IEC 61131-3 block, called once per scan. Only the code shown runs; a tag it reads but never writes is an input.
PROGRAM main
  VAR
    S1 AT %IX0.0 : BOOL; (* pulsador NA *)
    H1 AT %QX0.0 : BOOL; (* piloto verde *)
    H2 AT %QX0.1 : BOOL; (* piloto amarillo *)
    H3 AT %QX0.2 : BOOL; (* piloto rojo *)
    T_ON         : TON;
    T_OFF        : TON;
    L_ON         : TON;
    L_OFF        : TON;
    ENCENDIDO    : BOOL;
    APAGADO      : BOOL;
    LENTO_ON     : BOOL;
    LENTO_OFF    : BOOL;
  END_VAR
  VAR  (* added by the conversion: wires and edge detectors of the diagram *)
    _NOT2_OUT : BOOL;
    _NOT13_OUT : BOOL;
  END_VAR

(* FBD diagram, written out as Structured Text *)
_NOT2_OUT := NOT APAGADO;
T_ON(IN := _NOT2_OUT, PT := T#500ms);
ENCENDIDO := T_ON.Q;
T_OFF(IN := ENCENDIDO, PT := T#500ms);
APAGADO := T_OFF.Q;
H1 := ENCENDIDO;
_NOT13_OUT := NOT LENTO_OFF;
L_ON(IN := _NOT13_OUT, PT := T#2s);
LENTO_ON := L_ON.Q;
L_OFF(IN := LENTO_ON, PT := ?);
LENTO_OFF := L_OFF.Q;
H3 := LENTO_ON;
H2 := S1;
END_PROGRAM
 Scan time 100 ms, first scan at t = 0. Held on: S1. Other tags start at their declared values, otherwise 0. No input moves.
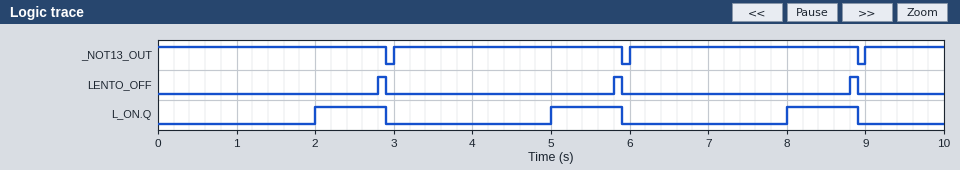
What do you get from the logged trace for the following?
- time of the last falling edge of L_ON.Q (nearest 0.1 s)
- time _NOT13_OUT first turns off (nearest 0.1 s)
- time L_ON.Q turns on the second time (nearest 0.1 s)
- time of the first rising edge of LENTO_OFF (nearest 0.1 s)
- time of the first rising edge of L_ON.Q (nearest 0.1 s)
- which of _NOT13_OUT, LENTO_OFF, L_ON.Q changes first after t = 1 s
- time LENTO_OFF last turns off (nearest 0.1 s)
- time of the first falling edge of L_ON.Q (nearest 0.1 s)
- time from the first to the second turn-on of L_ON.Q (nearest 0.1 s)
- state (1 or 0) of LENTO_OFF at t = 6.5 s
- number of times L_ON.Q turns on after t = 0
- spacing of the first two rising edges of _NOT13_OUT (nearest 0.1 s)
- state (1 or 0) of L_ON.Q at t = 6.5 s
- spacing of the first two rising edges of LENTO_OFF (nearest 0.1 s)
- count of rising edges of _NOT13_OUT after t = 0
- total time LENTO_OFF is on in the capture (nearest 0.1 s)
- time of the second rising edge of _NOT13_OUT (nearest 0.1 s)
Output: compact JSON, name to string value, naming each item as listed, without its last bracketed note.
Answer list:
{"time of the last falling edge of L_ON.Q": "8.9 s", "time _NOT13_OUT first turns off": "2.9 s", "time L_ON.Q turns on the second time": "5.0 s", "time of the first rising edge of LENTO_OFF": "2.8 s", "time of the first rising edge of L_ON.Q": "2.0 s", "which of _NOT13_OUT, LENTO_OFF, L_ON.Q changes first after t = 1 s": "L_ON.Q", "time LENTO_OFF last turns off": "8.9 s", "time of the first falling edge of L_ON.Q": "2.9 s", "time from the first to the second turn-on of L_ON.Q": "3.0 s", "state (1 or 0) of LENTO_OFF at t = 6.5 s": "0", "number of times L_ON.Q turns on after t = 0": "3", "spacing of the first two rising edges of _NOT13_OUT": "3.0 s", "state (1 or 0) of L_ON.Q at t = 6.5 s": "0", "spacing of the first two rising edges of LENTO_OFF": "3.0 s", "count of rising edges of _NOT13_OUT after t = 0": "3", "total time LENTO_OFF is on in the capture": "0.3 s", "time of the second rising edge of _NOT13_OUT": "6.0 s"}
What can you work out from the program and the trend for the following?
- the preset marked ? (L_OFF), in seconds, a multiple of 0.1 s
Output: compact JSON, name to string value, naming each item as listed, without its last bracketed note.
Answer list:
{"the preset marked ? (L_OFF), in seconds, a multiple of 0.1 s": "0.8 s"}
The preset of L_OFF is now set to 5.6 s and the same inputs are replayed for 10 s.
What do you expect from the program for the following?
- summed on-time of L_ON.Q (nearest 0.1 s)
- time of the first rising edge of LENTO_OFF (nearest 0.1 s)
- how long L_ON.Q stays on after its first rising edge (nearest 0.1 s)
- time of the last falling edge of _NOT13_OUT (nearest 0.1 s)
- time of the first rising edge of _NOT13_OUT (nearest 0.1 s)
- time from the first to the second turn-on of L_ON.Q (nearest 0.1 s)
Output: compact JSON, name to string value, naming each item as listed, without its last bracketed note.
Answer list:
{"summed on-time of L_ON.Q": "5.9 s", "time of the first rising edge of LENTO_OFF": "7.6 s", "how long L_ON.Q stays on after its first rising edge": "5.7 s", "time of the last falling edge of _NOT13_OUT": "7.7 s", "time of the first rising edge of _NOT13_OUT": "7.8 s", "time from the first to the second turn-on of L_ON.Q": "7.8 s"}
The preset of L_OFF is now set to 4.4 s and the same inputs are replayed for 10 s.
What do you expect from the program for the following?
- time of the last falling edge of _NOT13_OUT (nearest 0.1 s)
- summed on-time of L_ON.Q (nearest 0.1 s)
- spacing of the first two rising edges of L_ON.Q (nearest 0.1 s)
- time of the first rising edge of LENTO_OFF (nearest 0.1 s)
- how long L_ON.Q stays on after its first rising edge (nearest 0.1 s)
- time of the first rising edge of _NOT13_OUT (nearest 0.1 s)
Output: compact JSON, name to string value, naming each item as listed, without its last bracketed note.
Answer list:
{"time of the last falling edge of _NOT13_OUT": "6.5 s", "summed on-time of L_ON.Q": "5.9 s", "spacing of the first two rising edges of L_ON.Q": "6.6 s", "time of the first rising edge of LENTO_OFF": "6.4 s", "how long L_ON.Q stays on after its first rising edge": "4.5 s", "time of the first rising edge of _NOT13_OUT": "6.6 s"}
